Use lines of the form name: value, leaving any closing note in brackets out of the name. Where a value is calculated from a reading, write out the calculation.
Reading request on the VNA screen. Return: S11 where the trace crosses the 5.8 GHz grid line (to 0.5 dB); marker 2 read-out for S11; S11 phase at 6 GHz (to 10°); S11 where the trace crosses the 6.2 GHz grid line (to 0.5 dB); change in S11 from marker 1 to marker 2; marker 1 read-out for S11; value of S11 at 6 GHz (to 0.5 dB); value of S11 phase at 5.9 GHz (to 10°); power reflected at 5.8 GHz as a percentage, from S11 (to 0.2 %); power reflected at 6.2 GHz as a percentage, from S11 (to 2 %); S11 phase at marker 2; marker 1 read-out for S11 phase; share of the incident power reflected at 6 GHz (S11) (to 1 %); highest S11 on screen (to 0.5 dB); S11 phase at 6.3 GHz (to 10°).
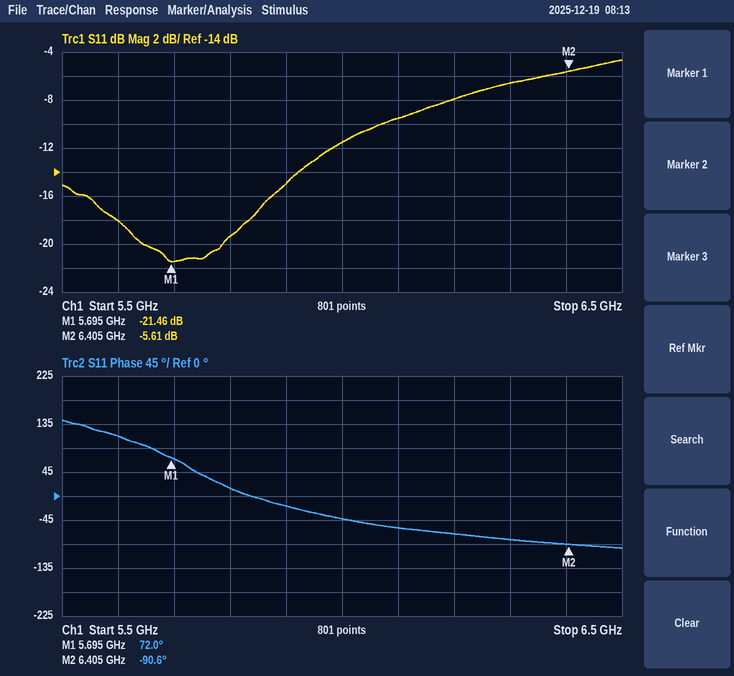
S11 where the trace crosses the 5.8 GHz grid line: -19.5 dB
marker 2 read-out for S11: -5.61 dB
S11 phase at 6 GHz: -40°
S11 where the trace crosses the 6.2 GHz grid line: -8.0 dB
change in S11 from marker 1 to marker 2: -5.61 − (-21.46) = 15.85 dB
marker 1 read-out for S11: -21.46 dB
value of S11 at 6 GHz: -11.5 dB
value of S11 phase at 5.9 GHz: -20°
power reflected at 5.8 GHz as a percentage, from S11: 10^(-19.5/10) ≈ 1.12 %, so 1.2 % to the nearest 0.2 %
power reflected at 6.2 GHz as a percentage, from S11: 10^(-8/10) ≈ 16 %
S11 phase at marker 2: -90.6°
marker 1 read-out for S11 phase: 72.0°
share of the incident power reflected at 6 GHz (S11): 10^(-11.5/10) ≈ 7 %
highest S11 on screen: -4.5 dB
S11 phase at 6.3 GHz: -80°
